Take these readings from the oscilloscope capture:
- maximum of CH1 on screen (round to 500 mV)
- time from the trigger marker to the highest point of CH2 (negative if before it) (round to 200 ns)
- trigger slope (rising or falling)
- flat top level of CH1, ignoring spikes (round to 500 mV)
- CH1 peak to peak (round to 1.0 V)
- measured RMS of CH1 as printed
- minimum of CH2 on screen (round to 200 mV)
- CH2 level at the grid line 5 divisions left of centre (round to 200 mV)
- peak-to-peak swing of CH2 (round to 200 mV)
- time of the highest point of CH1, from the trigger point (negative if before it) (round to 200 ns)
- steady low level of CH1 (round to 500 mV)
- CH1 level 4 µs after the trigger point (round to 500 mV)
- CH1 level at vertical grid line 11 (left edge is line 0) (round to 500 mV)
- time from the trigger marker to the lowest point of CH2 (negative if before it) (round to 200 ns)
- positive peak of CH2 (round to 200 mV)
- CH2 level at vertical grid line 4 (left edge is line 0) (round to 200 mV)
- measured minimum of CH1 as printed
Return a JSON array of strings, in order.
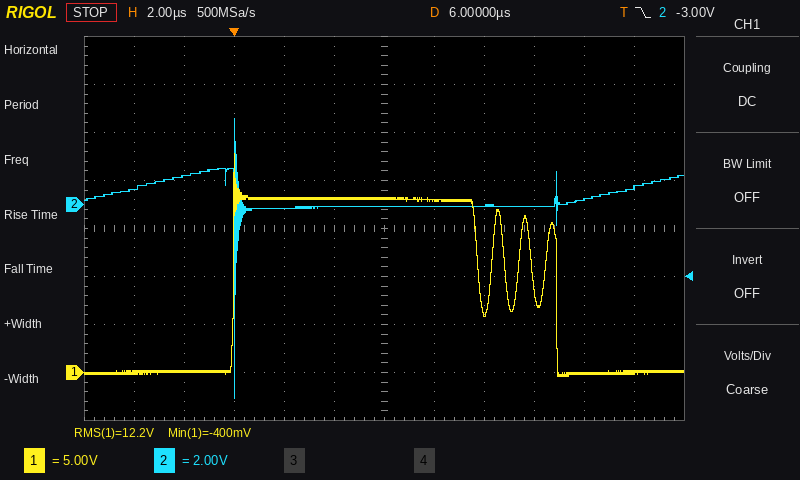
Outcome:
["23.0 V", "0.0 µs", "falling", "18.0 V", "23.0 V", "12.2 V", "-8.0 V", "600 mV", "11.6 V", "0.0 µs", "0.0 V", "18.0 V", "0.0 V", "0.0 µs", "3.6 V", "-200 mV", "-400 mV"]
